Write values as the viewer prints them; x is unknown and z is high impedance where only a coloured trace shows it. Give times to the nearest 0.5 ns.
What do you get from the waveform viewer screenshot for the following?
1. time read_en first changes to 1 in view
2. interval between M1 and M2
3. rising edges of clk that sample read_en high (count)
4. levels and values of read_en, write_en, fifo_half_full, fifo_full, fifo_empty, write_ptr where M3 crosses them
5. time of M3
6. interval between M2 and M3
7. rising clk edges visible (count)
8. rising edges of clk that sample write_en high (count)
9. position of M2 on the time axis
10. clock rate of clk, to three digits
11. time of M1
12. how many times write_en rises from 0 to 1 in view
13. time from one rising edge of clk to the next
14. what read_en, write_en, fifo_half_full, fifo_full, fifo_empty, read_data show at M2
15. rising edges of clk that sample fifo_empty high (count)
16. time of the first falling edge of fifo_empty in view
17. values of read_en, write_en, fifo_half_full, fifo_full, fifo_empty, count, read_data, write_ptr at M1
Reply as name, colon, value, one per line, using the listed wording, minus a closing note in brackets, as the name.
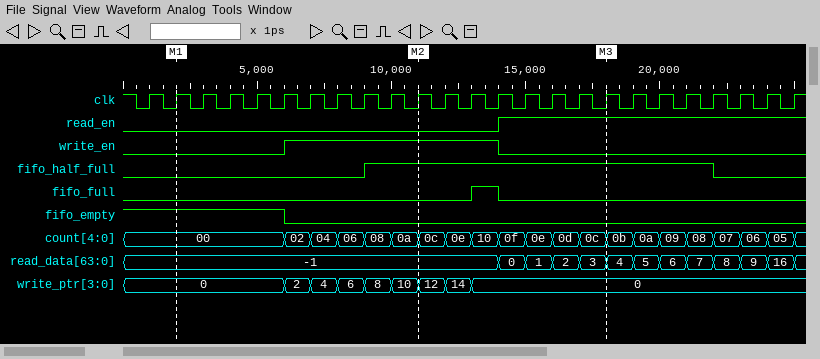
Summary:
time read_en first changes to 1 in view: 14 ns
interval between M1 and M2: 9 ns
rising edges of clk that sample read_en high: 11
levels and values of read_en, write_en, fifo_half_full, fifo_full, fifo_empty, write_ptr where M3 crosses them: read_en=1, write_en=0, fifo_half_full=1, fifo_full=0, fifo_empty=0, write_ptr=0
time of M3: 18 ns
interval between M2 and M3: 7 ns
rising clk edges visible: 25
rising edges of clk that sample write_en high: 8
position of M2 on the time axis: 11 ns
clock rate of clk, to three digits: 1.00 GHz
time of M1: 2 ns
how many times write_en rises from 0 to 1 in view: 1
time from one rising edge of clk to the next: 1 ns
what read_en, write_en, fifo_half_full, fifo_full, fifo_empty, read_data show at M2: read_en=0, write_en=1, fifo_half_full=1, fifo_full=0, fifo_empty=0, read_data=-1
rising edges of clk that sample fifo_empty high: 6
time of the first falling edge of fifo_empty in view: 6 ns
values of read_en, write_en, fifo_half_full, fifo_full, fifo_empty, count, read_data, write_ptr at M1: read_en=0, write_en=0, fifo_half_full=0, fifo_full=0, fifo_empty=1, count=00, read_data=-1, write_ptr=0
